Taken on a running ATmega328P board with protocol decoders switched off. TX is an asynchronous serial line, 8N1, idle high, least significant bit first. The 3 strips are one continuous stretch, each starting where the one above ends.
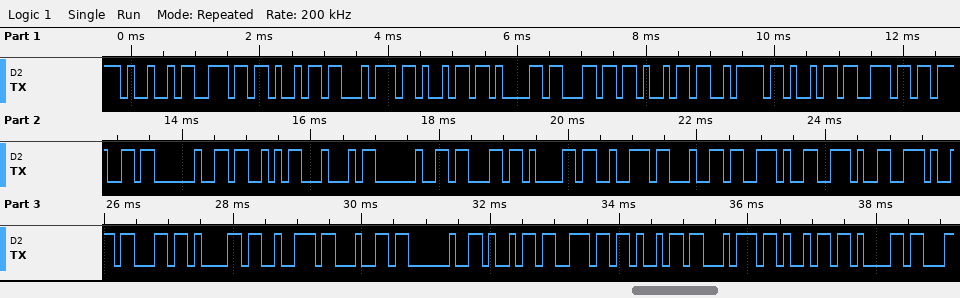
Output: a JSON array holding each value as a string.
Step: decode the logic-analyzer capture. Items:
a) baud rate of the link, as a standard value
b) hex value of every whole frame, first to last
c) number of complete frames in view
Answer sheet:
["9600 baud", "49 6E 69 74 69 61 6C 69 7A 69 6E 67 20 53 44 20 63 61 72 64 2E 2E 2E 63 61 72 64 20 69 6E 69 74 69 61", "34"]
